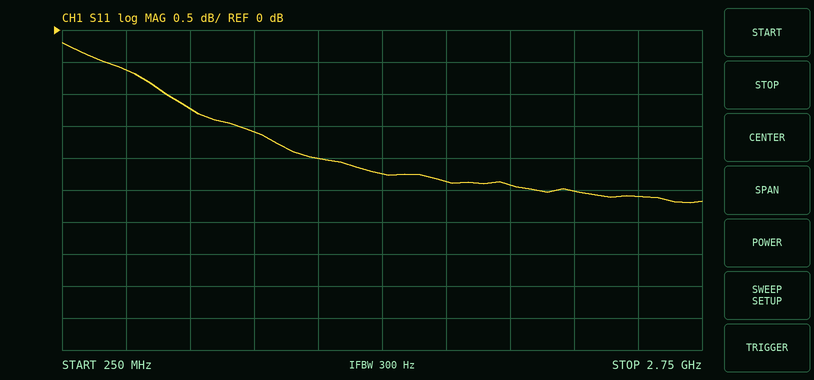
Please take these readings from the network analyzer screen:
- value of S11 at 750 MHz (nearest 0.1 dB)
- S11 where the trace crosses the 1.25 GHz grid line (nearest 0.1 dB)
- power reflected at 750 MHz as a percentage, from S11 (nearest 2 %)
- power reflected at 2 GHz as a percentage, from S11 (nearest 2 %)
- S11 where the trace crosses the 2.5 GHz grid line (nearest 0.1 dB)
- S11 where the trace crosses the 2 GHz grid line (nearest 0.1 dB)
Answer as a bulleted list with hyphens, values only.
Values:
- -1.2 dB
- -2.0 dB
- 76 %
- 58 %
- -2.6 dB
- -2.4 dB
